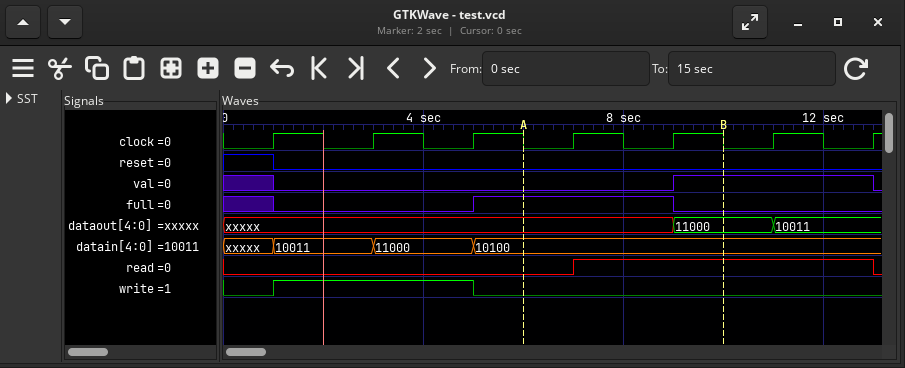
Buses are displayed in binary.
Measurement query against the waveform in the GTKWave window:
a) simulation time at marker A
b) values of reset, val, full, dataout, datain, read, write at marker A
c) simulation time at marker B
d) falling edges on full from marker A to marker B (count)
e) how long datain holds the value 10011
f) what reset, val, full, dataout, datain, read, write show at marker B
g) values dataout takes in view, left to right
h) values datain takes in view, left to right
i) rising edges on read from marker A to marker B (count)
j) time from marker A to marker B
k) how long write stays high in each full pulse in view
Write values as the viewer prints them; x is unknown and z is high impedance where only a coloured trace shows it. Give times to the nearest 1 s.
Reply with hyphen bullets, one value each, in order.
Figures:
- 6 s
- reset=0, val=0, full=1, dataout=xxxxx, datain=10100, read=0, write=0
- 10 s
- 1
- 2 s
- reset=0, val=1, full=0, dataout=11000, datain=10100, read=1, write=0
- xxxxx, 11000, 10011
- xxxxx, 10011, 11000, 10100
- 1
- 4 s
- 4 s
